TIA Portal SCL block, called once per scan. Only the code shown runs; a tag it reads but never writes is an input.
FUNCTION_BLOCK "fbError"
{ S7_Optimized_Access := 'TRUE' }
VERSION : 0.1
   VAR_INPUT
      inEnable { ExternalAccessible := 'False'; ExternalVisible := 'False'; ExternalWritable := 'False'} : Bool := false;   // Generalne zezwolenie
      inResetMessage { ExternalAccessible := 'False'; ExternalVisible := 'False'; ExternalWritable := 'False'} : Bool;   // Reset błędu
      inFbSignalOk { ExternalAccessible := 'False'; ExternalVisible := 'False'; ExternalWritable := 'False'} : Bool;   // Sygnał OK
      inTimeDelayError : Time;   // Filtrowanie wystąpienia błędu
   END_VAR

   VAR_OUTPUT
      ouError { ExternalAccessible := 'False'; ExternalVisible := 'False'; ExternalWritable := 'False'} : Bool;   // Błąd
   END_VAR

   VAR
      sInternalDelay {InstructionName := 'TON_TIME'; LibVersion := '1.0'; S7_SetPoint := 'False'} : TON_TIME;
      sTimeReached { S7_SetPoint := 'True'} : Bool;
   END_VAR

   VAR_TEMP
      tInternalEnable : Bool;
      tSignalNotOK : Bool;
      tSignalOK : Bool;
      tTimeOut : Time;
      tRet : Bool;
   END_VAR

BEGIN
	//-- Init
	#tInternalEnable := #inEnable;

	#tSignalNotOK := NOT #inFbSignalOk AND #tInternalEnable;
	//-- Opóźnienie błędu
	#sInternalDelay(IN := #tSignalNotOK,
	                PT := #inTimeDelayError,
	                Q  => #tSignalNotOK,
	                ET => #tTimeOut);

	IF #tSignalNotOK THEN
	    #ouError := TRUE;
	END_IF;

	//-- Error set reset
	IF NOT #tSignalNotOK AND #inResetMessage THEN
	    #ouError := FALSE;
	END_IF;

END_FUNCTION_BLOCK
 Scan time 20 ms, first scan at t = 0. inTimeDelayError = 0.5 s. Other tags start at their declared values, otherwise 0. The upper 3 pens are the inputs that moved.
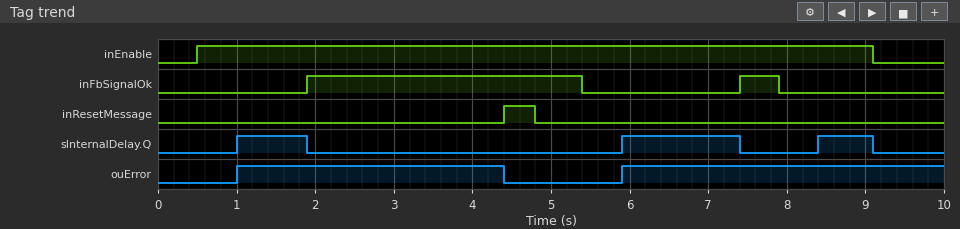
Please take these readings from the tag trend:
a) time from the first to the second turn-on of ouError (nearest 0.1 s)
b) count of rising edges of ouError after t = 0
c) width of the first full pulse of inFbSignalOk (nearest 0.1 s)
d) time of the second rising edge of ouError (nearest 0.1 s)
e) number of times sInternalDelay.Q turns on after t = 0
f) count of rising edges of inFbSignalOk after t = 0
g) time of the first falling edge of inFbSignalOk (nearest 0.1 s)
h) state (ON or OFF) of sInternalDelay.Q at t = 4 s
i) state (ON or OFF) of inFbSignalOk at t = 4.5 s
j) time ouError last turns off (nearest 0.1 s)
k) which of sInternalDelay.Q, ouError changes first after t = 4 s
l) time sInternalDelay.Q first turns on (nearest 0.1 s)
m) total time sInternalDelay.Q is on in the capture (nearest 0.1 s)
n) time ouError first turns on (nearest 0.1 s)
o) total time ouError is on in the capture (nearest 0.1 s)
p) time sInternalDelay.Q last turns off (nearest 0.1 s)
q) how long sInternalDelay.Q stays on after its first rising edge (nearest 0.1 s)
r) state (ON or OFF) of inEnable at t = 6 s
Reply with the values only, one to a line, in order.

4.9 s
2
3.5 s
5.9 s
3
2
5.4 s
OFF
ON
4.4 s
ouError
1.0 s
3.1 s
1.0 s
7.5 s
9.1 s
0.9 s
ON
